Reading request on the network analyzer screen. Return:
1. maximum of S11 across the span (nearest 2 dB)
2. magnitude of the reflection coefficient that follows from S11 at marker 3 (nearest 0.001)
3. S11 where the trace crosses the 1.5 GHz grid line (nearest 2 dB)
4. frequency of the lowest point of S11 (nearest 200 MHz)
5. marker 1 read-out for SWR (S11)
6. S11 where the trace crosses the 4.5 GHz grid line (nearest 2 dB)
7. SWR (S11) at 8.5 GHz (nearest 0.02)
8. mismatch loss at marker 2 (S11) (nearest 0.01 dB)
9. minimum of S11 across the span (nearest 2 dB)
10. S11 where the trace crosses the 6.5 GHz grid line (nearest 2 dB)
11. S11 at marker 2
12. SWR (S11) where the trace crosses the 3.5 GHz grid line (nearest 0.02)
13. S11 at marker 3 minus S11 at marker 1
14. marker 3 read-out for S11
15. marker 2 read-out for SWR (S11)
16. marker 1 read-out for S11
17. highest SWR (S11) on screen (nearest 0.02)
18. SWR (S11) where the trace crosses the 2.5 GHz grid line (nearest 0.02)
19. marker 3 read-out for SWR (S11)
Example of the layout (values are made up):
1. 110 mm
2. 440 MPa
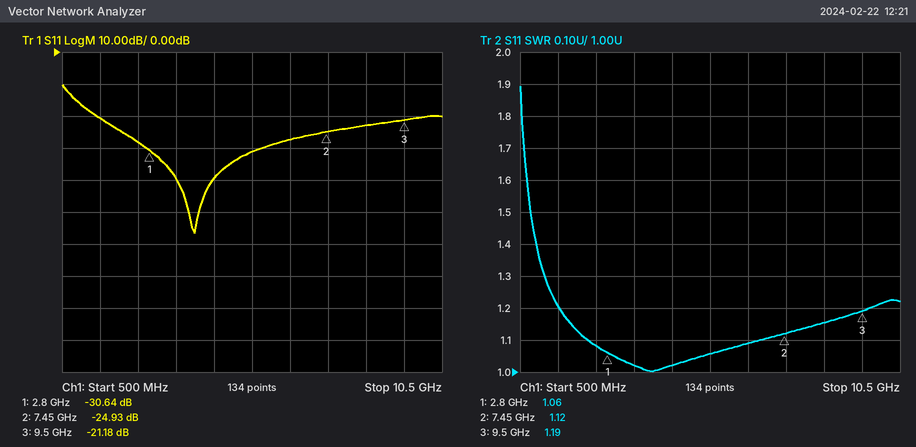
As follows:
1. -10 dB
2. 0.087
3. -20 dB
4. 4.0 GHz
5. 1.06
6. -40 dB
7. 1.16
8. 0.01 dB
9. -56 dB
10. -28 dB
11. -24.93 dB
12. 1.02
13. 9.46 dB
14. -21.18 dB
15. 1.12
16. -30.64 dB
17. 1.90
18. 1.08
19. 1.19
